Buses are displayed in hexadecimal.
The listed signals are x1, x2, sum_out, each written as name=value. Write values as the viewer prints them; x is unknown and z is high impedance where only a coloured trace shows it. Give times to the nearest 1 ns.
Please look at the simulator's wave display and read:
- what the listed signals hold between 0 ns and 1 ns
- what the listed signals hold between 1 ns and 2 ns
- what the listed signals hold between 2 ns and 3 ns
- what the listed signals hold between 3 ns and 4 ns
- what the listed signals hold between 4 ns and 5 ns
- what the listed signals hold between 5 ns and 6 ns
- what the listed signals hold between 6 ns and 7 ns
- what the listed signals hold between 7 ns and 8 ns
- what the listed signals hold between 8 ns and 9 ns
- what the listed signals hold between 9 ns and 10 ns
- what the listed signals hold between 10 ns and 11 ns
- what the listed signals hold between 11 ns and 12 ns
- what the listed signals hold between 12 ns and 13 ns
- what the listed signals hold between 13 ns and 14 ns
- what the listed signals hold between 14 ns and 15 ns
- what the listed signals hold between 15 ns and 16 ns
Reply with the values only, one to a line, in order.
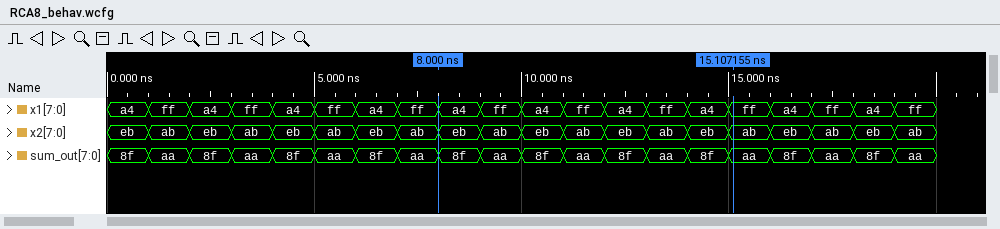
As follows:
x1=a4, x2=eb, sum_out=8f
x1=ff, x2=ab, sum_out=aa
x1=a4, x2=eb, sum_out=8f
x1=ff, x2=ab, sum_out=aa
x1=a4, x2=eb, sum_out=8f
x1=ff, x2=ab, sum_out=aa
x1=a4, x2=eb, sum_out=8f
x1=ff, x2=ab, sum_out=aa
x1=a4, x2=eb, sum_out=8f
x1=ff, x2=ab, sum_out=aa
x1=a4, x2=eb, sum_out=8f
x1=ff, x2=ab, sum_out=aa
x1=a4, x2=eb, sum_out=8f
x1=ff, x2=ab, sum_out=aa
x1=a4, x2=eb, sum_out=8f
x1=ff, x2=ab, sum_out=aa
